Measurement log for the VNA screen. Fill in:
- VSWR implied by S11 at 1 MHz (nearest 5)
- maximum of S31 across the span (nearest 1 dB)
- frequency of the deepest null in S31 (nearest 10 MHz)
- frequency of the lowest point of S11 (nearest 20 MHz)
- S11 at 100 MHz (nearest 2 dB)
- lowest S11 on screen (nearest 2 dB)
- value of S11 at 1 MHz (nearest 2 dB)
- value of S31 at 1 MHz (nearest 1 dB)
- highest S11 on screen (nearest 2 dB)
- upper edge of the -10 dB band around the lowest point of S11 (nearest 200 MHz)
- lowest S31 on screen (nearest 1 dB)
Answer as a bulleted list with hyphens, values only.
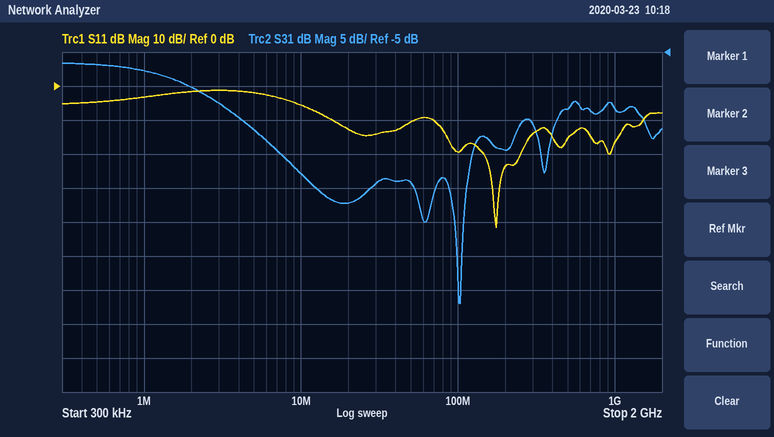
- 5
- -7 dB
- 100 MHz
- 180 MHz
- -20 dB
- -42 dB
- -4 dB
- -8 dB
- -2 dB
- 1.6 GHz
- -42 dB
